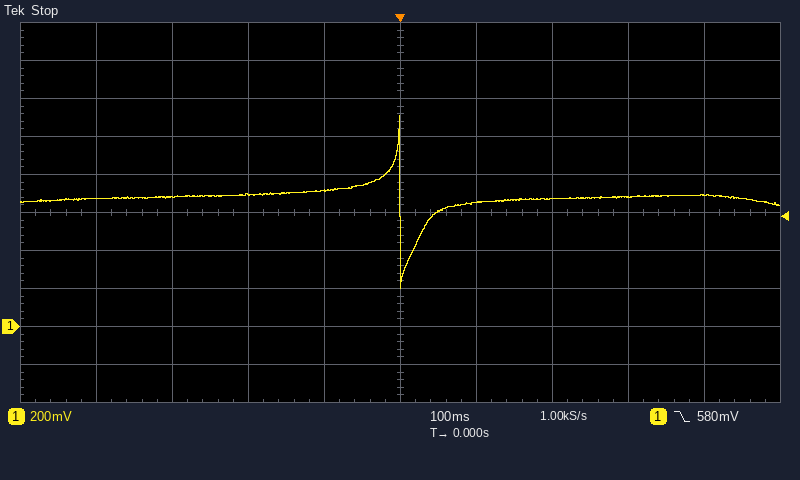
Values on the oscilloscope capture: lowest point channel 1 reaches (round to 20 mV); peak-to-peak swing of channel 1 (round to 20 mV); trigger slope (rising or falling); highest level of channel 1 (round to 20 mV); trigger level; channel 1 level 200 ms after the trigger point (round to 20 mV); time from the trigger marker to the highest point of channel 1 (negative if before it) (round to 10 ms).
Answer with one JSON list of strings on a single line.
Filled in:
["200 mV", "920 mV", "falling", "1.12 V", "580 mV", "680 mV", "0 ms"]
